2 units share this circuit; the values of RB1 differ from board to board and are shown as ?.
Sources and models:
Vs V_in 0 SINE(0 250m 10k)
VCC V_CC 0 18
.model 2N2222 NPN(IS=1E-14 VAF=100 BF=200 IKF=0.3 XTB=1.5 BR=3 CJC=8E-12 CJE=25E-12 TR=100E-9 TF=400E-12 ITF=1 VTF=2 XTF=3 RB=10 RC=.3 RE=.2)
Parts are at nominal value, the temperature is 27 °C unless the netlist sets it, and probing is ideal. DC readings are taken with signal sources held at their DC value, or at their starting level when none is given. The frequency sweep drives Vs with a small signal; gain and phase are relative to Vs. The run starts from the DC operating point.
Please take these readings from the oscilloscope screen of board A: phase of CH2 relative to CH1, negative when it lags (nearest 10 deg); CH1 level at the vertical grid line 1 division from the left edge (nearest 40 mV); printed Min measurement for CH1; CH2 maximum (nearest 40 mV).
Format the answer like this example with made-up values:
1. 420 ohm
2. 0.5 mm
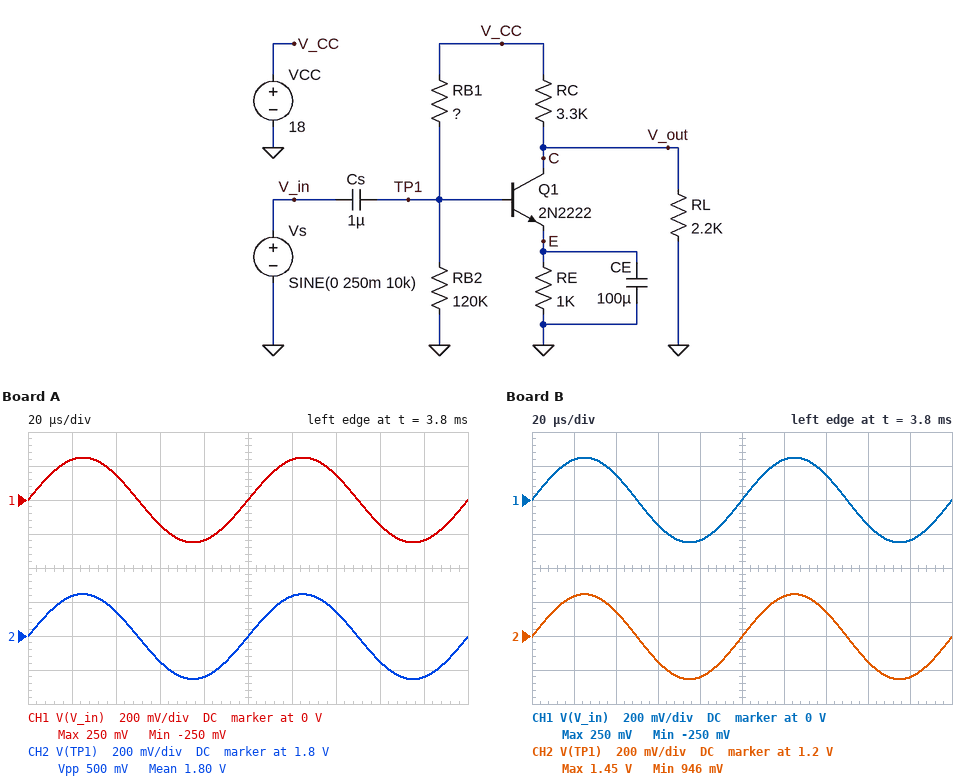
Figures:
1. 0 deg
2. 240 mV
3. -250 mV
4. 2.04 V
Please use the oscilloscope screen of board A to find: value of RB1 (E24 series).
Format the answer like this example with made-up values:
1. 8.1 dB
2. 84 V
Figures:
1. 680 kΩ
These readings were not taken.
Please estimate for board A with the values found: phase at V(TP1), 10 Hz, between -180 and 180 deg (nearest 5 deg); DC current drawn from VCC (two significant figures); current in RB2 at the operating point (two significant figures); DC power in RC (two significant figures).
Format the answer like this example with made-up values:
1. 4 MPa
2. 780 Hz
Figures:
1. 10 deg
2. 3.8 mA
3. 17 µA
4. 48 mW
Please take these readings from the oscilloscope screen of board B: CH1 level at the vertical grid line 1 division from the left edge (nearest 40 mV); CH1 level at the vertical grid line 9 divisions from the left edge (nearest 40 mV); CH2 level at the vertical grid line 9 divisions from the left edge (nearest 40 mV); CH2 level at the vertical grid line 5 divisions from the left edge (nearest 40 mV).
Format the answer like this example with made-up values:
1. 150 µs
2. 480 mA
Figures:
1. 240 mV
2. -240 mV
3. 960 mV
4. 1.20 V
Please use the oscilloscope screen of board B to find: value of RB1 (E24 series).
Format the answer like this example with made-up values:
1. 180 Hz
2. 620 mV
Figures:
1. 1.1 MΩ
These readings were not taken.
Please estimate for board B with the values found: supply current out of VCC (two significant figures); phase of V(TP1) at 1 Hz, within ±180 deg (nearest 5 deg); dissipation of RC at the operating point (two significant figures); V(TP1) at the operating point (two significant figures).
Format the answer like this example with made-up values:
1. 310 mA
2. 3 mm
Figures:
1. 3.6 mA
2. 55 deg
3. 42 mW
4. 1.4 V
